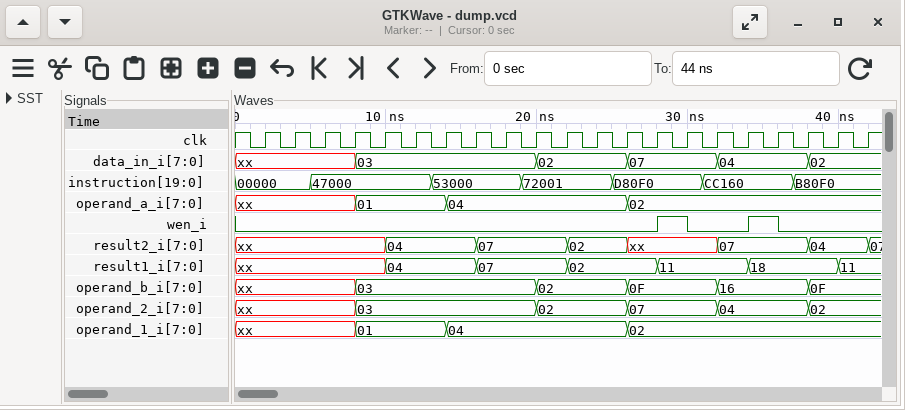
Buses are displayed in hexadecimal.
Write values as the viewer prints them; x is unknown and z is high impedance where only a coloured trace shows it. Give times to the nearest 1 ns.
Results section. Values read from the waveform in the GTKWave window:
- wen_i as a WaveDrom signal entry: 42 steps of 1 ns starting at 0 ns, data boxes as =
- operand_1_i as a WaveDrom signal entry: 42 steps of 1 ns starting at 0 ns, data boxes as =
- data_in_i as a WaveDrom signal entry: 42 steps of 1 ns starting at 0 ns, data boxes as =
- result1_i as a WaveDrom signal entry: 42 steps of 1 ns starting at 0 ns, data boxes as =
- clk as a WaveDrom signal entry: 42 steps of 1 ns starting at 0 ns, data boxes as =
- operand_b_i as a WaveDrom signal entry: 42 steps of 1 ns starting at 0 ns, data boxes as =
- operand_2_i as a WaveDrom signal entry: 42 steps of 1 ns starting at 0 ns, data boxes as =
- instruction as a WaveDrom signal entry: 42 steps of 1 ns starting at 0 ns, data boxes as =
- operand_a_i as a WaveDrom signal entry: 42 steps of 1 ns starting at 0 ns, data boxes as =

{name: 'wen_i', wave: '0...........................1.0...1.0.....'}
{name: 'operand_1_i', wave: 'x.......=.....=...........=...............', data: '01 04 02'}
{name: 'data_in_i', wave: 'x.......=...........=.....=.....=.....=...', data: '03 02 07 04 02'}
{name: 'result1_i', wave: 'x.........=.....=.....=.....=.....=.....=.', data: '04 07 02 11 18 11'}
{name: 'clk', wave: '101010101010101010101010101010101010101010'}
{name: 'operand_b_i', wave: 'x.......=...........=.....=.....=.....=...', data: '03 02 0F 16 0F'}
{name: 'operand_2_i', wave: 'x.......=...........=.....=.....=.....=...', data: '03 02 07 04 02'}
{name: 'instruction', wave: '=....=.......=.....=.....=.....=.....=....', data: '00000 47000 53000 72001 D80F0 CC160 B80F0'}
{name: 'operand_a_i', wave: 'x.......=.....=...........=...............', data: '01 04 02'}
